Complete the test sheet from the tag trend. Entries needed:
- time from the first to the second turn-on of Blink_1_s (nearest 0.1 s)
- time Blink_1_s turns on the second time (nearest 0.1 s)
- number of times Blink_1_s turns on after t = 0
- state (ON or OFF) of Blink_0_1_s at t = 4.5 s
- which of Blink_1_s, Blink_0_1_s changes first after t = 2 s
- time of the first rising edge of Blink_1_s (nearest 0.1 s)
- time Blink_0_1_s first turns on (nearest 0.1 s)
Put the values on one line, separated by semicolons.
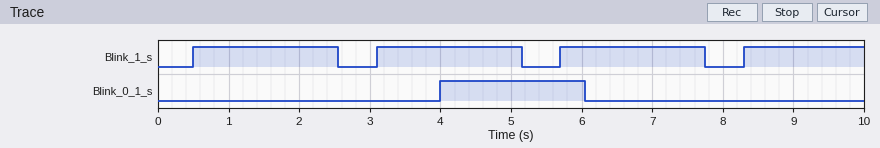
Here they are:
2.6 s; 3.1 s; 4; ON; Blink_1_s; 0.5 s; 4.0 s
